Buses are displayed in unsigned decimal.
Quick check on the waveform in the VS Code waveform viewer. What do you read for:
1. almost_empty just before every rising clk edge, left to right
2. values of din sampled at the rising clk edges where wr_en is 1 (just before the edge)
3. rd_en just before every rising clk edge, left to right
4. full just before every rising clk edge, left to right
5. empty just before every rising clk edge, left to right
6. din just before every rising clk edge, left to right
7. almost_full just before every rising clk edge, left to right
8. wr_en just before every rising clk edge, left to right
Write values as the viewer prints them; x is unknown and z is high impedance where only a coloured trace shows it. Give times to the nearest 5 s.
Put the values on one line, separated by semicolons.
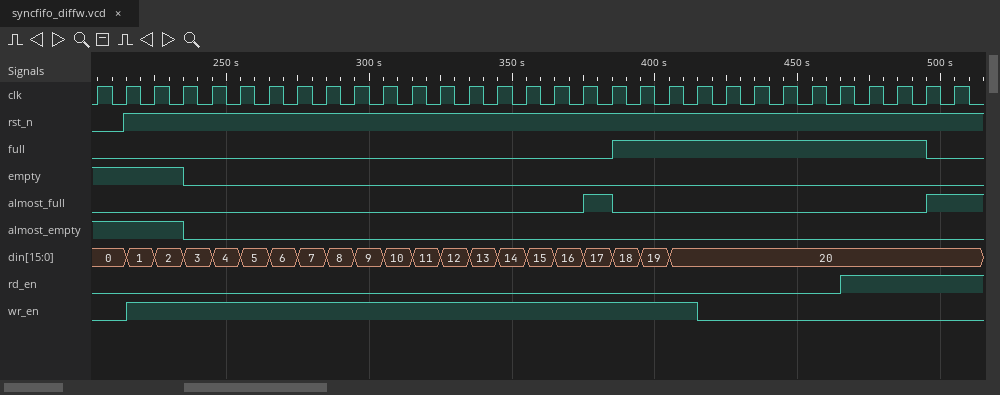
1 1 1 1 0 0 0 0 0 0 0 0 0 0 0 0 0 0 0 0 0 0 0 0 0 0 0 0 0 0 0; 1, 2, 3, 4, 5, 6, 7, 8, 9, 10, 11, 12, 13, 14, 15, 16, 17, 18, 19, 20; 0 0 0 0 0 0 0 0 0 0 0 0 0 0 0 0 0 0 0 0 0 0 0 0 0 0 0 1 1 1 1; 0 0 0 0 0 0 0 0 0 0 0 0 0 0 0 0 0 0 0 1 1 1 1 1 1 1 1 1 1 1 0; 1 1 1 1 0 0 0 0 0 0 0 0 0 0 0 0 0 0 0 0 0 0 0 0 0 0 0 0 0 0 0; 0, 0, 1, 2, 3, 4, 5, 6, 7, 8, 9, 10, 11, 12, 13, 14, 15, 16, 17, 18, 19, 20, 20, 20, 20, 20, 20, 20, 20, 20, 20; 0 0 0 0 0 0 0 0 0 0 0 0 0 0 0 0 0 0 1 0 0 0 0 0 0 0 0 0 0 0 1; 0 0 1 1 1 1 1 1 1 1 1 1 1 1 1 1 1 1 1 1 1 1 0 0 0 0 0 0 0 0 0
